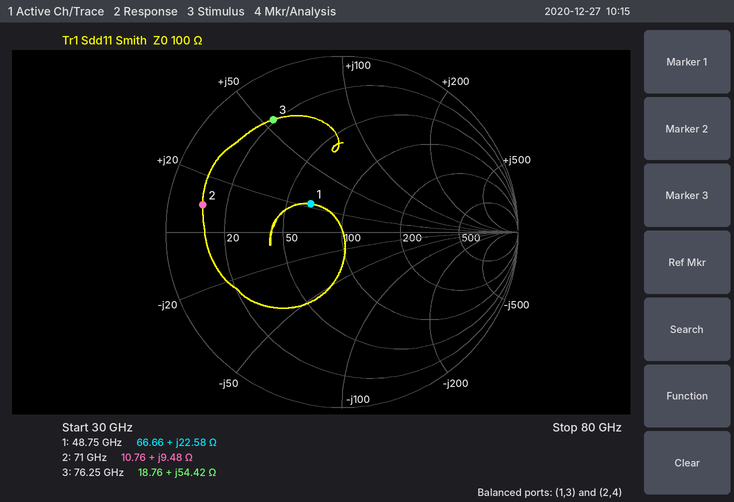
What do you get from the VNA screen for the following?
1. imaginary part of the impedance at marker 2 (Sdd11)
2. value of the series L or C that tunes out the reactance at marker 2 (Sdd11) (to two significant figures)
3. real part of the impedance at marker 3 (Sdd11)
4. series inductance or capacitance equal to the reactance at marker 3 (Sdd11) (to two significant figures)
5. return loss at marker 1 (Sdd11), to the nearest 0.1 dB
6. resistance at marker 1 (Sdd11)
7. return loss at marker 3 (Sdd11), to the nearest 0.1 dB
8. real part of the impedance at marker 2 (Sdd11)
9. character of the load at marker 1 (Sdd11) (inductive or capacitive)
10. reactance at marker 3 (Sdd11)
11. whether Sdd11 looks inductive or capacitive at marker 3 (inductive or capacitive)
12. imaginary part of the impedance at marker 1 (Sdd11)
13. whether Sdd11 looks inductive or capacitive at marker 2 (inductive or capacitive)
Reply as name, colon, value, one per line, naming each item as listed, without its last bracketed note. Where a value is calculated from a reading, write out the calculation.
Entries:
imaginary part of the impedance at marker 2: +9.48 Ω
value of the series L or C that tunes out the reactance at marker 2 (Sdd11): C = 1/(2π × 71 GHz × 9.48 Ω) ≈ 236 fF, so 240 fF to two significant figures
real part of the impedance at marker 3: 18.76 Ω
series inductance or capacitance equal to the reactance at marker 3 (Sdd11): L = 54.42 Ω/(2π × 76.25 GHz) ≈ 114 pH, so 110 pH to two significant figures
return loss at marker 1 (Sdd11), to the nearest 0.1 dB: 12.4 dB
resistance at marker 1: 66.66 Ω
return loss at marker 3 (Sdd11), to the nearest 0.1 dB: 2.5 dB
real part of the impedance at marker 2: 10.76 Ω
character of the load at marker 1 (Sdd11): inductive
reactance at marker 3: +54.42 Ω
whether Sdd11 looks inductive or capacitive at marker 3: inductive
imaginary part of the impedance at marker 1: +22.58 Ω
whether Sdd11 looks inductive or capacitive at marker 2: inductive
